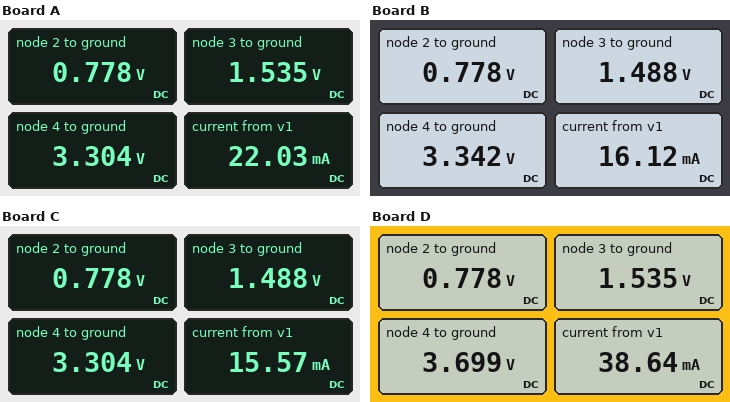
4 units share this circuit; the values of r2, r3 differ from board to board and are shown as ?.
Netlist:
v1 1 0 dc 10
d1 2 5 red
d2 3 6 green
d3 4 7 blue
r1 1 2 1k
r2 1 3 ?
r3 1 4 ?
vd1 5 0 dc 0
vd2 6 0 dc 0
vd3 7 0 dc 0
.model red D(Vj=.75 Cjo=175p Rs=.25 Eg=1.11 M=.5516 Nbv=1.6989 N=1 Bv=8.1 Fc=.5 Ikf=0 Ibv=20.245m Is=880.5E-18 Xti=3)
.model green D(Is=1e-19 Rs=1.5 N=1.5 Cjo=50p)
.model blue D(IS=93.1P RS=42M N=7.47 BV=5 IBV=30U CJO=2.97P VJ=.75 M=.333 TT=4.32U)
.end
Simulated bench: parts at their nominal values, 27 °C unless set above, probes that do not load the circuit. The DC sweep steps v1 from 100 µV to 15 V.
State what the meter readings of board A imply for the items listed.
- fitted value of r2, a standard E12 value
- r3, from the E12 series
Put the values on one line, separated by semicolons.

820 Ω; 2.7 kΩ
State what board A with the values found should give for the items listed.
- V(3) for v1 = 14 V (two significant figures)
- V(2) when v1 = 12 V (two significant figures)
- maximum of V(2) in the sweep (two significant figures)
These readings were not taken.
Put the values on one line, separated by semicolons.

1.6 V; 780 mV; 790 mV
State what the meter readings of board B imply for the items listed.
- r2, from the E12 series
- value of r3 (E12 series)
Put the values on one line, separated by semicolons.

2.2 kΩ; 2.2 kΩ
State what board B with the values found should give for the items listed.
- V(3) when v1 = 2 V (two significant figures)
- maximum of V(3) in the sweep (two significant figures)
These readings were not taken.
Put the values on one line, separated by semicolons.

1.4 V; 1.5 V
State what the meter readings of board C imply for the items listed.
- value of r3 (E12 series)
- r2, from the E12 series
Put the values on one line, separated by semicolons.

2.7 kΩ; 2.2 kΩ
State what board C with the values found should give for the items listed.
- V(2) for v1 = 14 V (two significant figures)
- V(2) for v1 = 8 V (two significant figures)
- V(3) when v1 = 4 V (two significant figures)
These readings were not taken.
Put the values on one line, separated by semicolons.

790 mV; 770 mV; 1.4 V
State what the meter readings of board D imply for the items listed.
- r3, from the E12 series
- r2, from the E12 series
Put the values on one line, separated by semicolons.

330 Ω; 820 Ω
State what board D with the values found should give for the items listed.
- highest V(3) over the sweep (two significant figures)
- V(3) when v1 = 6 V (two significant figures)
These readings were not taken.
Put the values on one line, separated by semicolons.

1.6 V; 1.5 V
